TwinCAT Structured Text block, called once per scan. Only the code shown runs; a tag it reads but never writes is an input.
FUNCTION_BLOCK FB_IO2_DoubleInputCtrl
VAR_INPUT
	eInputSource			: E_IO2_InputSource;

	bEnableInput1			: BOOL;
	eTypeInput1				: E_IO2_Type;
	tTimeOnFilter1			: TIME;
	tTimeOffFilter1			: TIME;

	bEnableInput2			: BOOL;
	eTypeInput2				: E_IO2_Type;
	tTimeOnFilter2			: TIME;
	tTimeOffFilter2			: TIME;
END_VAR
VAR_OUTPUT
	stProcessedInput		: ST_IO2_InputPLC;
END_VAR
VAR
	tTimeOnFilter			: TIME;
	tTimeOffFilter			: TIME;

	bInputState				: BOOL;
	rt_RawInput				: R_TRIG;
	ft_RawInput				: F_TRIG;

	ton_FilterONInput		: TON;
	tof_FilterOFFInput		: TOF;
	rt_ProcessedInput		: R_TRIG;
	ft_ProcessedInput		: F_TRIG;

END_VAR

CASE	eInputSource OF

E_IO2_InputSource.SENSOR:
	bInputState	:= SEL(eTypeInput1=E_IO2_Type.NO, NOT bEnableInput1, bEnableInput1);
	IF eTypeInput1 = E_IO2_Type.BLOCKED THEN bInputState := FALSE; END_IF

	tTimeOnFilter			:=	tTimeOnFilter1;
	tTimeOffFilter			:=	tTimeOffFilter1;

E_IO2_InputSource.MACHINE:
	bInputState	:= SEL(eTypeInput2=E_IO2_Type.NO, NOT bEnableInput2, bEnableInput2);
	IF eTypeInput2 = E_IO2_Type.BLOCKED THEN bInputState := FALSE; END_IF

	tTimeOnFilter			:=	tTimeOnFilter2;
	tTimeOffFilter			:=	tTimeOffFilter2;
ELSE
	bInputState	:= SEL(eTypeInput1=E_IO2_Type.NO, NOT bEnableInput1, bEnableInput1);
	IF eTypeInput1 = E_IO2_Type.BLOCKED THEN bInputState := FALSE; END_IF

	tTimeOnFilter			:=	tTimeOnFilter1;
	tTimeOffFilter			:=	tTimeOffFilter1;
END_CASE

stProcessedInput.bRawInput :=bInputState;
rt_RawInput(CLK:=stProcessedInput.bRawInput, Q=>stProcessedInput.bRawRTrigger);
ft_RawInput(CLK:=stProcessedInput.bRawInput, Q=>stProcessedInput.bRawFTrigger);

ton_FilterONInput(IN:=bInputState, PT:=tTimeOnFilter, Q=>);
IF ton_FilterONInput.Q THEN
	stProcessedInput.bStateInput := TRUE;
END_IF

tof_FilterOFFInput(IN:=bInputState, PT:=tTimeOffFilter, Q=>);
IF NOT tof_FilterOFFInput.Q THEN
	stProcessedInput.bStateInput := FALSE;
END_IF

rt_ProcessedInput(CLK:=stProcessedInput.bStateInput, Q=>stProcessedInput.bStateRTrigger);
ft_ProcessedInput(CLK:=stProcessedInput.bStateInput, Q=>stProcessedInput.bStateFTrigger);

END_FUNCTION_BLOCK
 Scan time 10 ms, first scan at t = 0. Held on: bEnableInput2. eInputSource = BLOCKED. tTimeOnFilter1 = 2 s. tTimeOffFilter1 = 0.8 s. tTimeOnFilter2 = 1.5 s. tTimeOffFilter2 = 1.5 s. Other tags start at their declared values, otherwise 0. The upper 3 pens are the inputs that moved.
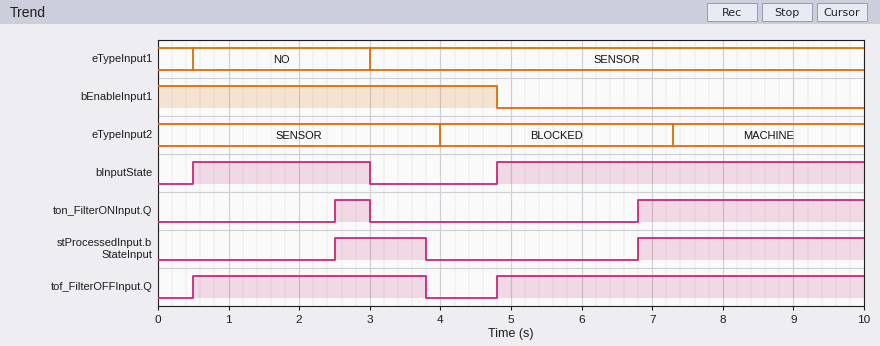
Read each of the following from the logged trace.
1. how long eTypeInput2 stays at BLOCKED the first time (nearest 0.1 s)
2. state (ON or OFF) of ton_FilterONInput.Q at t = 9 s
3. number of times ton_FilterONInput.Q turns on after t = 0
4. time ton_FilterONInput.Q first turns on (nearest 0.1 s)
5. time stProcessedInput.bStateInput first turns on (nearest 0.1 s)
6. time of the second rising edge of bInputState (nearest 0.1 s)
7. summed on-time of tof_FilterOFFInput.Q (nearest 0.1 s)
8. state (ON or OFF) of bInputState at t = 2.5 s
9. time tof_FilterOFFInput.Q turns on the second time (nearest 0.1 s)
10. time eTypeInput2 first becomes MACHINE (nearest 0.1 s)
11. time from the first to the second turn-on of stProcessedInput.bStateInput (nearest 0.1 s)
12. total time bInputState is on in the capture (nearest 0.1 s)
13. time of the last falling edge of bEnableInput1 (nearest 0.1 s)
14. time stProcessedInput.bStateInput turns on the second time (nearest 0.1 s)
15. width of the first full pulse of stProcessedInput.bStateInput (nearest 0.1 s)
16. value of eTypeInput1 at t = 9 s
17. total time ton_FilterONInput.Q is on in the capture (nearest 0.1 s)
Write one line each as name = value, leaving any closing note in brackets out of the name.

how long eTypeInput2 stays at BLOCKED the first time = 3.3 s
state (ON or OFF) of ton_FilterONInput.Q at t = 9 s = ON
number of times ton_FilterONInput.Q turns on after t = 0 = 2
time ton_FilterONInput.Q first turns on = 2.5 s
time stProcessedInput.bStateInput first turns on = 2.5 s
time of the second rising edge of bInputState = 4.8 s
summed on-time of tof_FilterOFFInput.Q = 8.5 s
state (ON or OFF) of bInputState at t = 2.5 s = ON
time tof_FilterOFFInput.Q turns on the second time = 4.8 s
time eTypeInput2 first becomes MACHINE = 7.3 s
time from the first to the second turn-on of stProcessedInput.bStateInput = 4.3 s
total time bInputState is on in the capture = 7.7 s
time of the last falling edge of bEnableInput1 = 4.8 s
time stProcessedInput.bStateInput turns on the second time = 6.8 s
width of the first full pulse of stProcessedInput.bStateInput = 1.3 s
value of eTypeInput1 at t = 9 s = SENSOR
total time ton_FilterONInput.Q is on in the capture = 3.7 s
